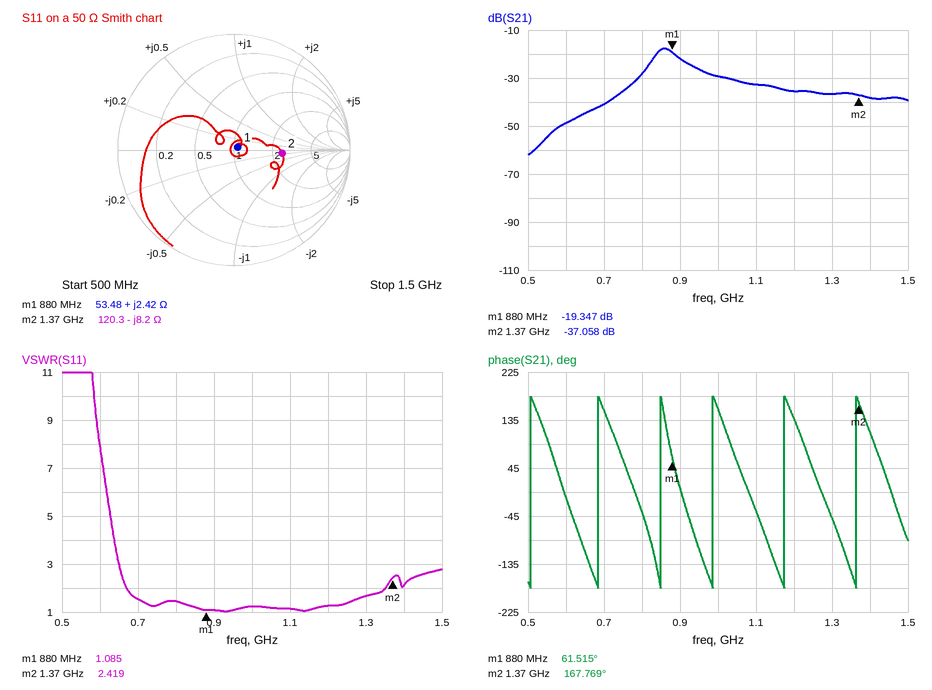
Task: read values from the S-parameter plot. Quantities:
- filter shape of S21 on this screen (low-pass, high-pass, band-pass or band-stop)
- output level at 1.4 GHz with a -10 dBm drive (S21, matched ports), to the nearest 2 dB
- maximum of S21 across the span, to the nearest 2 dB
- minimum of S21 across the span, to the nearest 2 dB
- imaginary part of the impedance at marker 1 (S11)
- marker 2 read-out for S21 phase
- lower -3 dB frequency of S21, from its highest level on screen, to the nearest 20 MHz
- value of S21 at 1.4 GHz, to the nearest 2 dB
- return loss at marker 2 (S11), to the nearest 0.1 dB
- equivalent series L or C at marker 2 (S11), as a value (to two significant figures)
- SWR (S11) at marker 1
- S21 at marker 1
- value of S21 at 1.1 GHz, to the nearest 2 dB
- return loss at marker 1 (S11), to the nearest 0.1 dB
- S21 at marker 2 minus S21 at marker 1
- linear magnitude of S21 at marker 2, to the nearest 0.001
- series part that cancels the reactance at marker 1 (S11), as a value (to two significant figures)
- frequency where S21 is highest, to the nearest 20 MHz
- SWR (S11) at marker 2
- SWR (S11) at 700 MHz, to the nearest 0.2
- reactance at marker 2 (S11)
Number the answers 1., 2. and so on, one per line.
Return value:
1. band-pass
2. -48 dBm
3. -18 dB
4. -62 dB
5. +2.42 Ω
6. 167.769°
7. 840 MHz
8. -38 dB
9. 7.6 dB
10. 14 pF
11. 1.085
12. -19.347 dB
13. -32 dB
14. 27.8 dB
15. -17.711 dB
16. 0.014
17. 75 pF
18. 860 MHz
19. 2.419
20. 1.6
21. -8.2 Ω
